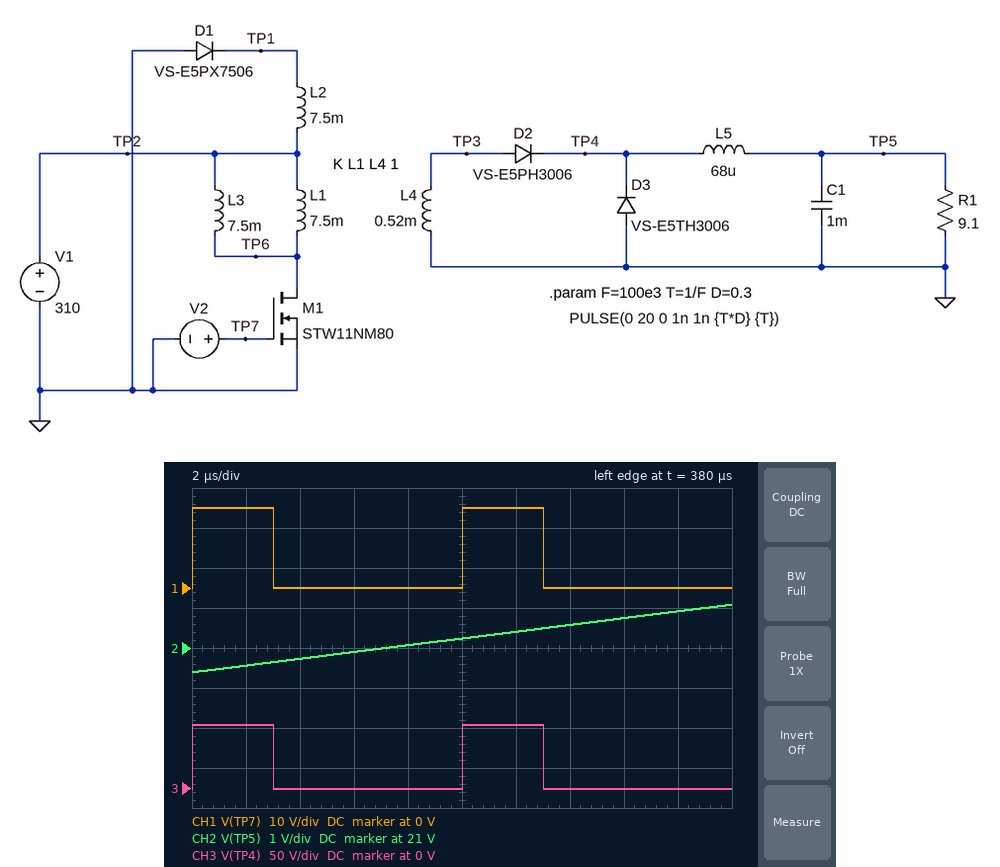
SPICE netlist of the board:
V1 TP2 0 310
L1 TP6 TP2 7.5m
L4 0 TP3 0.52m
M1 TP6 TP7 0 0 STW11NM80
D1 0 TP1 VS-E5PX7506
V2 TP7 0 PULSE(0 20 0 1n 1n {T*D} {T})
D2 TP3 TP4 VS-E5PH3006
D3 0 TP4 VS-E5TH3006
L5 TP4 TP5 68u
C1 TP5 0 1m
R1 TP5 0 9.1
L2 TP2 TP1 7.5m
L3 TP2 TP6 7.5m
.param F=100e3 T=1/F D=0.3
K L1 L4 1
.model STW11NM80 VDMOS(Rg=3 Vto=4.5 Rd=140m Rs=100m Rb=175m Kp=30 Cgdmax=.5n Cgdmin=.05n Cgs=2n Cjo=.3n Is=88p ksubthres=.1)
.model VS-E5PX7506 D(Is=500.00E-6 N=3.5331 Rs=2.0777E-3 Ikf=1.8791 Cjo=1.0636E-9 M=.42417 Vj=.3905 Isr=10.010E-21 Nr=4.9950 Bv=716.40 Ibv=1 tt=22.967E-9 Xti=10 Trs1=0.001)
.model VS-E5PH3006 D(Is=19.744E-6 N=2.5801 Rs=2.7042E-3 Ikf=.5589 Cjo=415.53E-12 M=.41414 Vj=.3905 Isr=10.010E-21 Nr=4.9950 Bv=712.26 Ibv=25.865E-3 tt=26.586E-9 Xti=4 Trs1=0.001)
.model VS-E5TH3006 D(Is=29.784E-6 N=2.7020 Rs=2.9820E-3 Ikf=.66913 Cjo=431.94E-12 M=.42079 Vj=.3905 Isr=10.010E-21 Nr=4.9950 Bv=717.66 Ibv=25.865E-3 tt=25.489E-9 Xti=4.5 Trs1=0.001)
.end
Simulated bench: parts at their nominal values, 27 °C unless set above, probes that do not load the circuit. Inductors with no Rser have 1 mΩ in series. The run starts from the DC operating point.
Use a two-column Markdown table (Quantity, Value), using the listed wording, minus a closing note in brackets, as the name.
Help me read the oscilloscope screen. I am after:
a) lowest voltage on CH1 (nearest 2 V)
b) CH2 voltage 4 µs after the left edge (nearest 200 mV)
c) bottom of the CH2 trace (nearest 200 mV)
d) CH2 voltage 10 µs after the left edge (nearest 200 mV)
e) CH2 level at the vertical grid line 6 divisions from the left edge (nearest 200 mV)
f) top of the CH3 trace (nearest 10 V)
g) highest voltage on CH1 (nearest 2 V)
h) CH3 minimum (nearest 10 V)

| Quantity | Value |
|---|---|
| lowest voltage on CH1 | 0 V |
| CH2 voltage 4 µs after the left edge | 20.8 V |
| bottom of the CH2 trace | 20.4 V |
| CH2 voltage 10 µs after the left edge | 21.2 V |
| CH2 level at the vertical grid line 6 divisions from the left edge | 21.4 V |
| top of the CH3 trace | 80 V |
| highest voltage on CH1 | 20 V |
| CH3 minimum | 0 V |
